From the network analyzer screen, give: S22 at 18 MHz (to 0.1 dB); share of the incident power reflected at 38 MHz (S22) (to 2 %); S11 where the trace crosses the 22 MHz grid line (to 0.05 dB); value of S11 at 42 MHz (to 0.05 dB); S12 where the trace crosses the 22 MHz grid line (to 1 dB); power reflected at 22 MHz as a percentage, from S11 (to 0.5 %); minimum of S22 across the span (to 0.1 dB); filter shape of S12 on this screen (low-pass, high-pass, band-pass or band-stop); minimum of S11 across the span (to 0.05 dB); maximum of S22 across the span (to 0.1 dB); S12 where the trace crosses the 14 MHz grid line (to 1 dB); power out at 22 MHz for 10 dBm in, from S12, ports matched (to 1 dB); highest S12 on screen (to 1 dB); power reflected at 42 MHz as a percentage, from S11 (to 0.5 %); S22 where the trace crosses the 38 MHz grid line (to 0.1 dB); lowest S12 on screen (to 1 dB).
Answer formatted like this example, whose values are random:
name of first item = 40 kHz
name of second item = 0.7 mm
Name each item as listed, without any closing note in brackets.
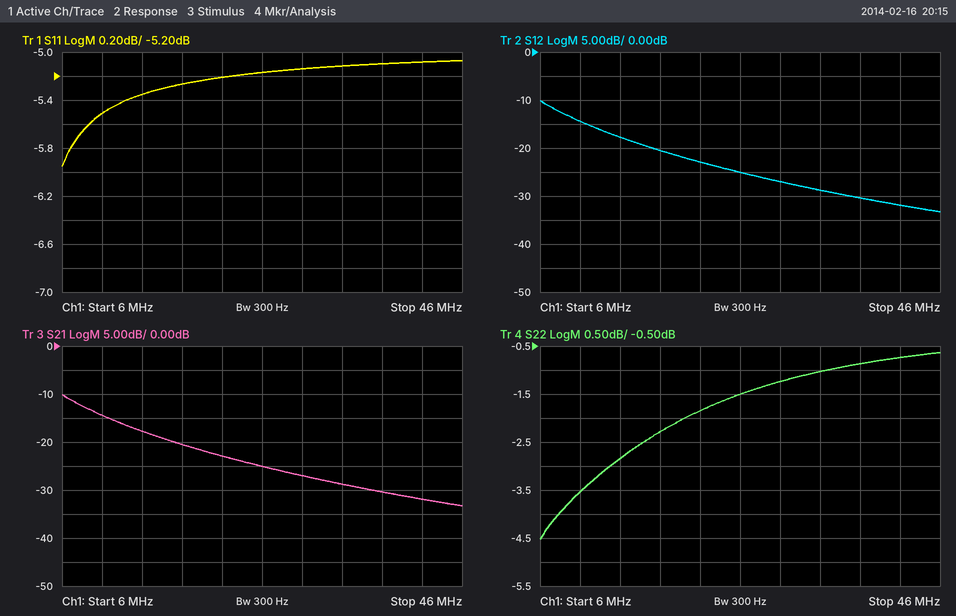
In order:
S22 at 18 MHz = -2.3 dB
share of the incident power reflected at 38 MHz (S22) = 82 %
S11 where the trace crosses the 22 MHz grid line = -5.20 dB
value of S11 at 42 MHz = -5.10 dB
S12 where the trace crosses the 22 MHz grid line = -23 dB
power reflected at 22 MHz as a percentage, from S11 = 30.0 %
minimum of S22 across the span = -4.5 dB
filter shape of S12 on this screen = low-pass
minimum of S11 across the span = -5.95 dB
maximum of S22 across the span = -0.6 dB
S12 where the trace crosses the 14 MHz grid line = -18 dB
power out at 22 MHz for 10 dBm in, from S12, ports matched = -13 dBm
highest S12 on screen = -10 dB
power reflected at 42 MHz as a percentage, from S11 = 31.0 %
S22 where the trace crosses the 38 MHz grid line = -0.9 dB
lowest S12 on screen = -33 dB
